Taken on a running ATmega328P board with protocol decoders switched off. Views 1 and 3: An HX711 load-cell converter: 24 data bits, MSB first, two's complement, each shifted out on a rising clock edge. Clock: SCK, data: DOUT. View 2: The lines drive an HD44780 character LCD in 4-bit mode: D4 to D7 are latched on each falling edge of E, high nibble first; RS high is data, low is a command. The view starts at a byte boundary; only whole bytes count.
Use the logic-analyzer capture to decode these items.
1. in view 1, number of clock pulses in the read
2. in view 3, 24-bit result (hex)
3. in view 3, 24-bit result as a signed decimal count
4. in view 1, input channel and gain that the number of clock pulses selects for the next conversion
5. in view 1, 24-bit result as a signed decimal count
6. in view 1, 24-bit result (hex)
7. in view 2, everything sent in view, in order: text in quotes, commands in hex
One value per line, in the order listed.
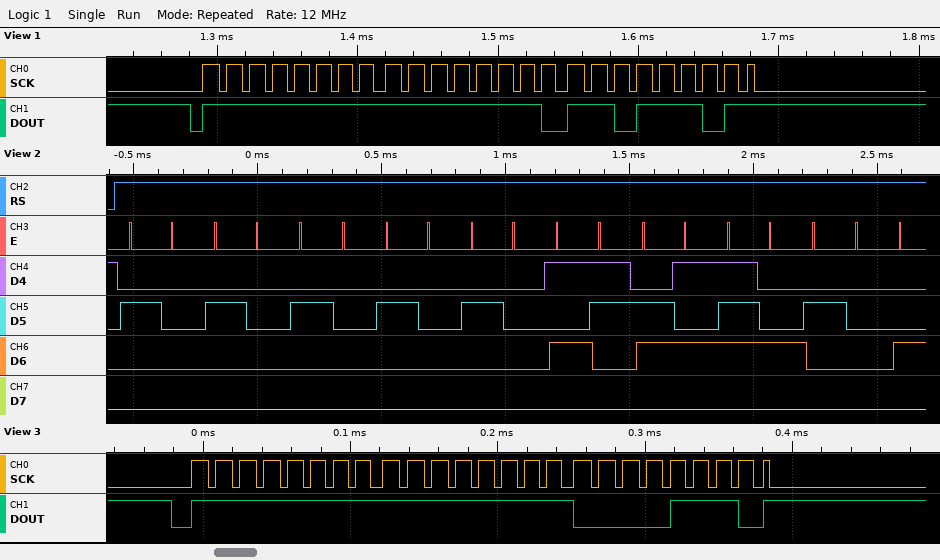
25
0xFFFF0E
-242
channel A, gain 128
-291
0xFFFEDD
"     Set "
